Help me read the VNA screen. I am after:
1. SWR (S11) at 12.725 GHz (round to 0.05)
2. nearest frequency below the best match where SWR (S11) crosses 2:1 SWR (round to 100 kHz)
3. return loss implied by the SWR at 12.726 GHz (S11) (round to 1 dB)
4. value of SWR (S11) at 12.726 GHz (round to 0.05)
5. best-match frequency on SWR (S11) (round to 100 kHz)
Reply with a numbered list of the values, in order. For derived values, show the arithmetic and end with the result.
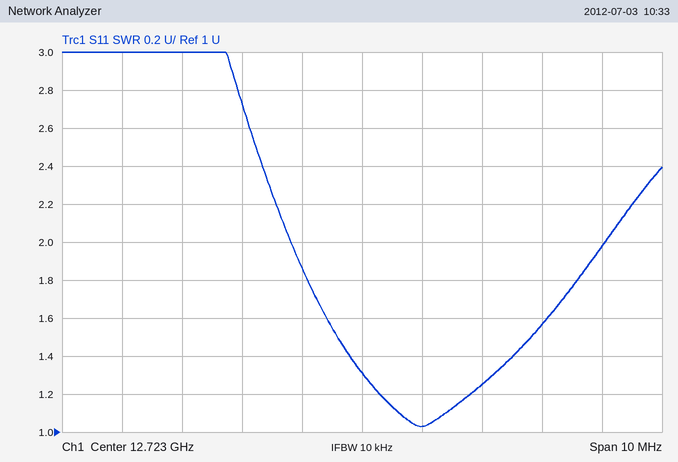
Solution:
1. 1.25
2. 12.7218 GHz
3. −20 log10((1.55 − 1)/(1.55 + 1)) ≈ 13 dB
4. 1.55
5. 12.7240 GHz
